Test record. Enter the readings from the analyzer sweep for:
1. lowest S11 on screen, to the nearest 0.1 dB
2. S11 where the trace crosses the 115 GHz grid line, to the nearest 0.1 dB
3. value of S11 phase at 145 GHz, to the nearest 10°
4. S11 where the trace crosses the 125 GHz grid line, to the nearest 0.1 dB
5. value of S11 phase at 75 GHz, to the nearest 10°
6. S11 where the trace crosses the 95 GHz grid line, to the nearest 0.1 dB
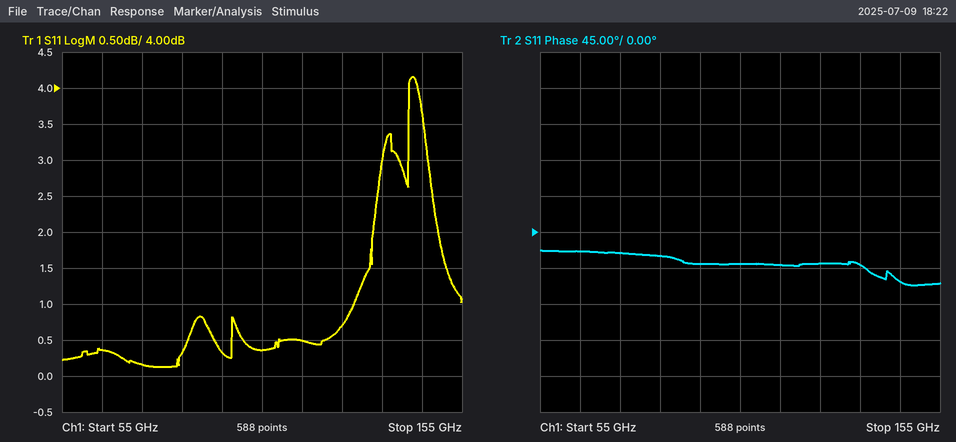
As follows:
0.1 dB
0.5 dB
-60°
0.7 dB
-30°
0.3 dB
